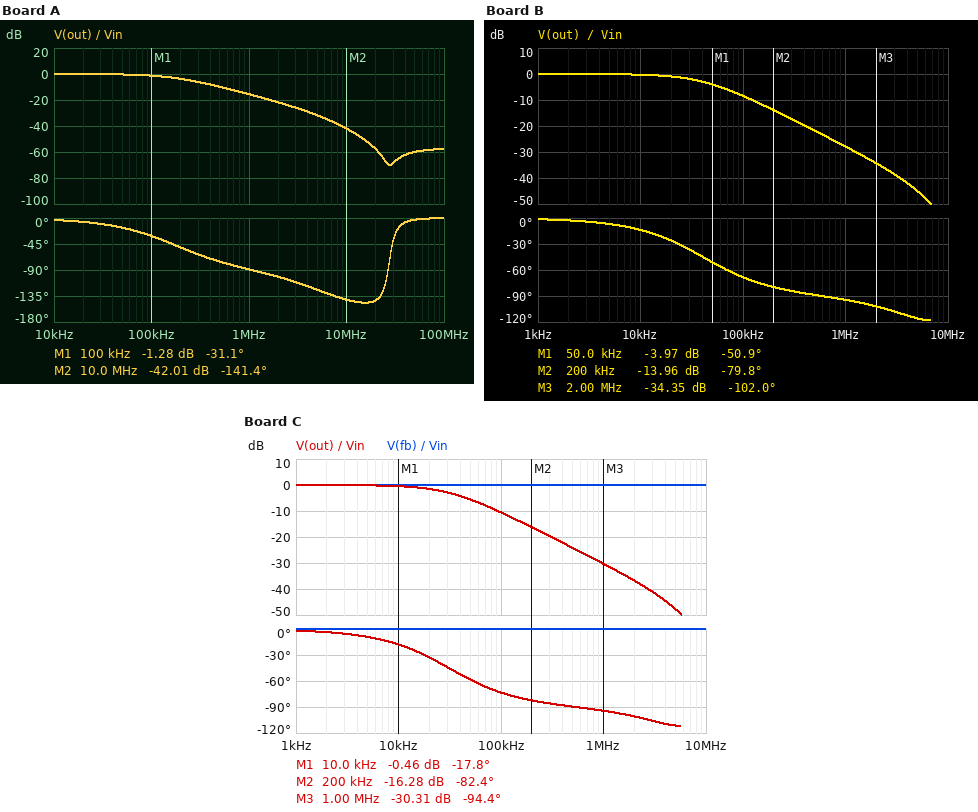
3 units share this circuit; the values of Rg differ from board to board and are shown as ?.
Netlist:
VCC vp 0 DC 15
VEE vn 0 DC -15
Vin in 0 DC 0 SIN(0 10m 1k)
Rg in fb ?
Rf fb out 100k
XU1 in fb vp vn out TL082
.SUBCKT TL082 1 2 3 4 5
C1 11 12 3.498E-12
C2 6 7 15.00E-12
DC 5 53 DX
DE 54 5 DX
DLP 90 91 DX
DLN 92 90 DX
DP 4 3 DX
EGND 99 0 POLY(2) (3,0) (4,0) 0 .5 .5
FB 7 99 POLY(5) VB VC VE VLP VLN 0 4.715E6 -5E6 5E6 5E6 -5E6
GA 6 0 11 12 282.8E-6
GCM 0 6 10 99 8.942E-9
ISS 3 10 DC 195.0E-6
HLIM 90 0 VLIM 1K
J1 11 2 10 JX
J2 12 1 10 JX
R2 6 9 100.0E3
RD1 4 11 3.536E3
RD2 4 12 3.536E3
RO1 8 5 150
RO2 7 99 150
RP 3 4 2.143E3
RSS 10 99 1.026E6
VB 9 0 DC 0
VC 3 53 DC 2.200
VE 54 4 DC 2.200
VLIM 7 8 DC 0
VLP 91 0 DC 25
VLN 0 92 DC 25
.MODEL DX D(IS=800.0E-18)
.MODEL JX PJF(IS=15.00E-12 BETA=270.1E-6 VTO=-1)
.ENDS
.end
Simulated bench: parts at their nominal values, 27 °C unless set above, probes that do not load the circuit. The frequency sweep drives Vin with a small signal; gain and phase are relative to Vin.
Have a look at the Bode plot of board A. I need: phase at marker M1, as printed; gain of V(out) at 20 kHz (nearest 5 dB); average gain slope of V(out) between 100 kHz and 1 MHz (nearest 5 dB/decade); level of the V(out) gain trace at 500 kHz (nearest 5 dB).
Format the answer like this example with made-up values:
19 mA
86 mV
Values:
-31.1 deg
0 dB
-15 dB/decade
-10 dB
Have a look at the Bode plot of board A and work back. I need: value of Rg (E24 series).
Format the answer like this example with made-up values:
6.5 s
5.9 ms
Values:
5.1 kΩ
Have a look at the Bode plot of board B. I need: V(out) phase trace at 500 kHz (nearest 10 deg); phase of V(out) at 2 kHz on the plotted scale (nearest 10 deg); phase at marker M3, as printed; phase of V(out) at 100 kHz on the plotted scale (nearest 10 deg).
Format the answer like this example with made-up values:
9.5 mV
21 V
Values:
-90 deg
0 deg
-102.0 deg
-70 deg
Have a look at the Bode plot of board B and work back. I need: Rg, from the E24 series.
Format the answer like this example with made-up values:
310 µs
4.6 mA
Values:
1.2 kΩ
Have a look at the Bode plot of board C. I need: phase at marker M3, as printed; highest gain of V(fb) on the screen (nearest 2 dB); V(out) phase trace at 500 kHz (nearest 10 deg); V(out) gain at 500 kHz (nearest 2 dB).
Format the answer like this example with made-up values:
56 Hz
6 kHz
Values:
-94.4 deg
0 dB
-90 deg
-24 dB
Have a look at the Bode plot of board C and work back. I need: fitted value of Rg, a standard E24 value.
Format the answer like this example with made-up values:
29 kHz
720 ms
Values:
910 Ω
